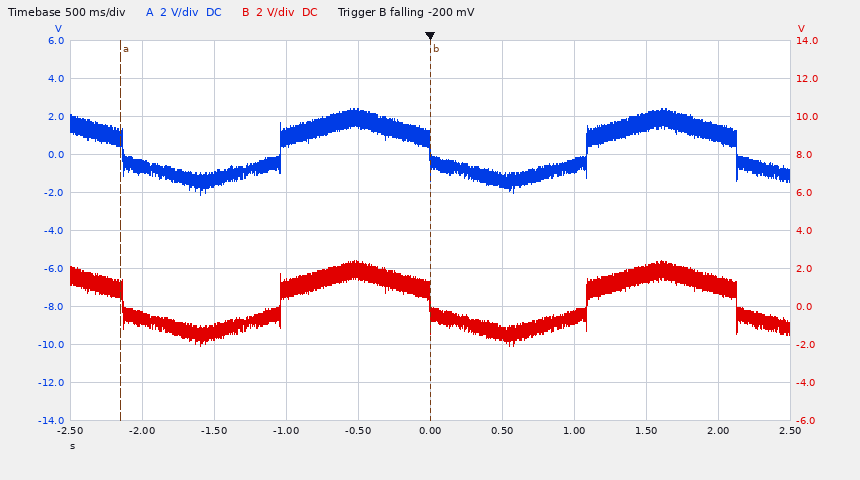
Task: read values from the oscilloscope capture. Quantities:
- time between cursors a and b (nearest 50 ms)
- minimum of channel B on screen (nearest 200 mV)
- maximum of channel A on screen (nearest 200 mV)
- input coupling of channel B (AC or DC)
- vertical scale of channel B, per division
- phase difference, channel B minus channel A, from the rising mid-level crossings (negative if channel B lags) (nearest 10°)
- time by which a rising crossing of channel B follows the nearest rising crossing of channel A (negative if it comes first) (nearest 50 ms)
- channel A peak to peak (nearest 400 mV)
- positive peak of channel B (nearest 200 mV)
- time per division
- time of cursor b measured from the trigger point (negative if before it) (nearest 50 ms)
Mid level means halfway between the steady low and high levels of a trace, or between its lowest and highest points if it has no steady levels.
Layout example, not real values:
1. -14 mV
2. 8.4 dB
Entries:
1. 2.15 s
2. -2.0 V
3. 2.4 V
4. DC
5. 2 V
6. 0°
7. 0 ms
8. 4.4 V
9. 2.4 V
10. 500 ms
11. 0 ms
